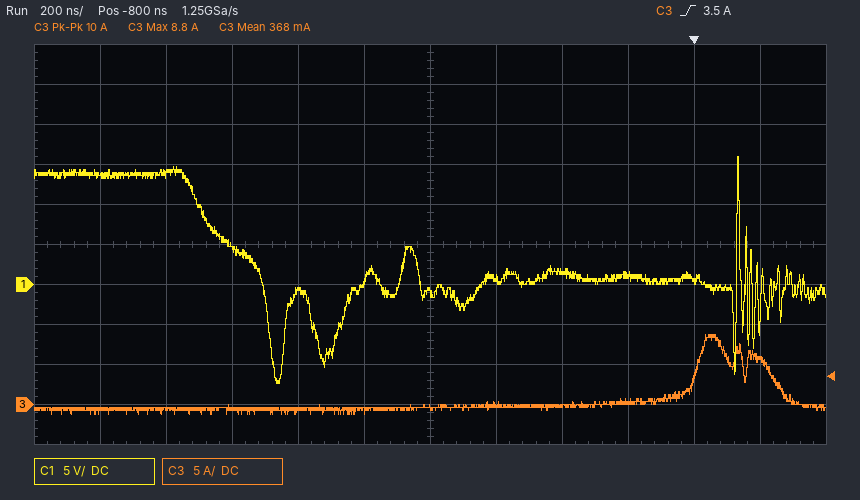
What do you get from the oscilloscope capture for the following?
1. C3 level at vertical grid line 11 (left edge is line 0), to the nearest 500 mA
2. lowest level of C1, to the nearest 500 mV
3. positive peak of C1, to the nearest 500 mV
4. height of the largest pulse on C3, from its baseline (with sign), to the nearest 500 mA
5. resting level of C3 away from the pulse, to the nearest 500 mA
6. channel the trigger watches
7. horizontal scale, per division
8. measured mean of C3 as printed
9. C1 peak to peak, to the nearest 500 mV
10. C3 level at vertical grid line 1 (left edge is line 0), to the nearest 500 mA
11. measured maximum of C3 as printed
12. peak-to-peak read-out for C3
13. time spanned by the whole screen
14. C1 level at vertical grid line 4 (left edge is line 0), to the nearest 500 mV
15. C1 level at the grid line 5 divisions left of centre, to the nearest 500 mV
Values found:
5.5 A
-12.5 V
16.0 V
+9.5 A
-500 mA
C3
200 ns
368 mA
28.5 V
-1.0 A
8.8 A
10 A
2.4 µs
-1.0 V
13.5 V
